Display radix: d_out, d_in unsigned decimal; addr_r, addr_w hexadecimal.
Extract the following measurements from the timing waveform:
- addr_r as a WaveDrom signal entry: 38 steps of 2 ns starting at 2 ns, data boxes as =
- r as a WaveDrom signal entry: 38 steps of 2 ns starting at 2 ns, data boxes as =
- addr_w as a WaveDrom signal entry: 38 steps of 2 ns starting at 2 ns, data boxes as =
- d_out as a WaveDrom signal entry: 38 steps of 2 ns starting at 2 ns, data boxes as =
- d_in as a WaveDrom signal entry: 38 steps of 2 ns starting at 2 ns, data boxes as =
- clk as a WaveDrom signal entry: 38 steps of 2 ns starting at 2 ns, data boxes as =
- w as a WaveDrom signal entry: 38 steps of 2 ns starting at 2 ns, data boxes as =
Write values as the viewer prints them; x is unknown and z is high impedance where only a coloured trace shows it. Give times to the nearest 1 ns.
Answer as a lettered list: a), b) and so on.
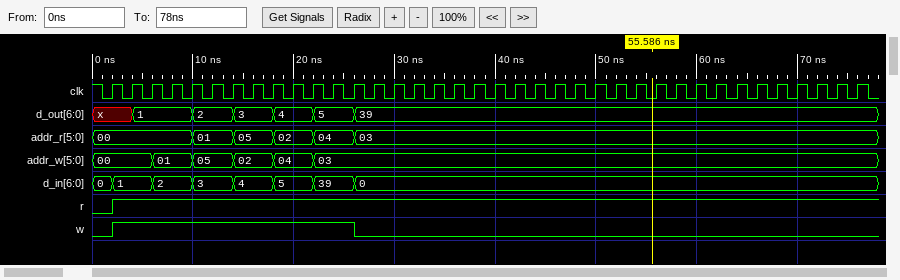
a) {name: 'addr_r', wave: '=...=.=.=.=.=.........................', data: '00 01 05 02 04 03'}
b) {name: 'r', wave: '1.....................................'}
c) {name: 'addr_w', wave: '=.=.=.=.=.=...........................', data: '00 01 05 02 04 03'}
d) {name: 'd_out', wave: 'x=..=.=.=.=.=.........................', data: '1 2 3 4 5 39'}
e) {name: 'd_in', wave: '=.=.=.=.=.=.=.........................', data: '1 2 3 4 5 39 0'}
f) {name: 'clk', wave: 'p.....................................'}
g) {name: 'w', wave: '1...........0.........................'}
